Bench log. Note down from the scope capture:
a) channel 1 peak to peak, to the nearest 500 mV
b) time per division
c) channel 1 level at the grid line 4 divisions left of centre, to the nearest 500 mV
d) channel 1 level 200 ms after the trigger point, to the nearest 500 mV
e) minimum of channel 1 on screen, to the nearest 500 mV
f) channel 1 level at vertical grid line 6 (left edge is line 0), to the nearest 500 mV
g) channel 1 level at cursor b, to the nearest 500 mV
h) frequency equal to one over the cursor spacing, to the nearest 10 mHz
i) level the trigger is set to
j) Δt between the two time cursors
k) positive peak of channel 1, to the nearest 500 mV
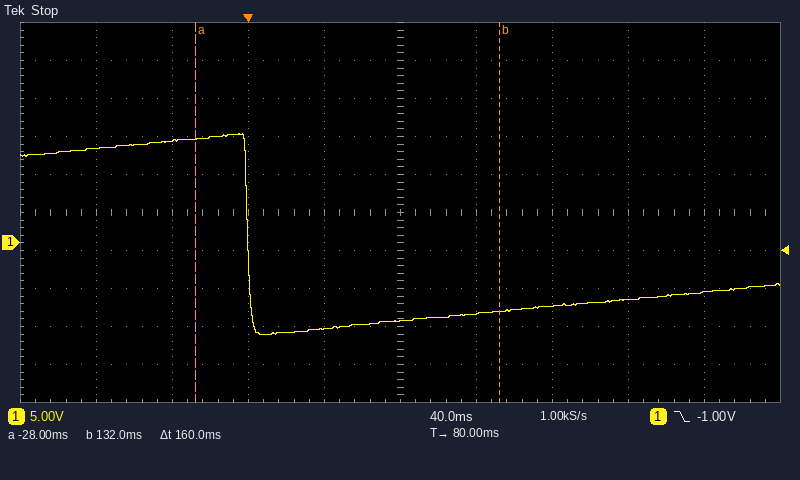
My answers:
26.5 V
40 ms
12.5 V
-7.5 V
-12.0 V
-9.5 V
-9.0 V
6.25 Hz
-1.00 V
160 ms
14.5 V
